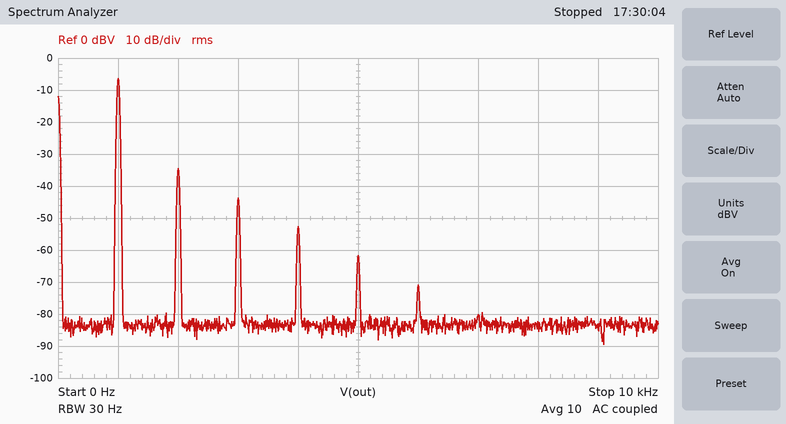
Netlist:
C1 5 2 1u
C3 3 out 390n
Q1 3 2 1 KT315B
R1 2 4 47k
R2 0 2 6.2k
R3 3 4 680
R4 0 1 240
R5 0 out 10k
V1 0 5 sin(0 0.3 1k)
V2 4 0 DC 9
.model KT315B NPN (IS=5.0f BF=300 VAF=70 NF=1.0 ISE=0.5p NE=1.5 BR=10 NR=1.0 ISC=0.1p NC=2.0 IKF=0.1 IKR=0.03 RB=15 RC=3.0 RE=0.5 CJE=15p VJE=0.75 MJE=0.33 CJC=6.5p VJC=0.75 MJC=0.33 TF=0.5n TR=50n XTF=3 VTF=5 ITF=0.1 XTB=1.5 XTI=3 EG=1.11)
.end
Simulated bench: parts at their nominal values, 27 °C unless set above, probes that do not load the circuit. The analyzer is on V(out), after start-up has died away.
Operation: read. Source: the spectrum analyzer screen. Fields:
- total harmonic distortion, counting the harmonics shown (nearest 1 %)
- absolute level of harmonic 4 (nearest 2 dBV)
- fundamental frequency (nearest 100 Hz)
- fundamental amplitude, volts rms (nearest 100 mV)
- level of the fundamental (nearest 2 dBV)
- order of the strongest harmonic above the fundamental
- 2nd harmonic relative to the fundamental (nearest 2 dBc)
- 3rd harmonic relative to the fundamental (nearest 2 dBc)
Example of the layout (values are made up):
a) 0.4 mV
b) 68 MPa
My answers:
a) 4 %
b) -52 dBV
c) 1.0 kHz
d) 500 mV
e) -6 dBV
f) 2
g) -28 dBc
h) -38 dBc
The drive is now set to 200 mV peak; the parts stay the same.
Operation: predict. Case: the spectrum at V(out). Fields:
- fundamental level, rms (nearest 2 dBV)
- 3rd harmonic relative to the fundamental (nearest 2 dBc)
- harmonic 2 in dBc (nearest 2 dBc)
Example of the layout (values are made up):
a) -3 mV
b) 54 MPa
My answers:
a) -10 dBV
b) -48 dBc
c) -34 dBc
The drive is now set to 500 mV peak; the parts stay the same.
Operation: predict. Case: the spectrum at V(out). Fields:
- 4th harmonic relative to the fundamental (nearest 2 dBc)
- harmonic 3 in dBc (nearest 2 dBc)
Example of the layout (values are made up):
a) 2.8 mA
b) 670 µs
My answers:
a) -34 dBc
b) -24 dBc
